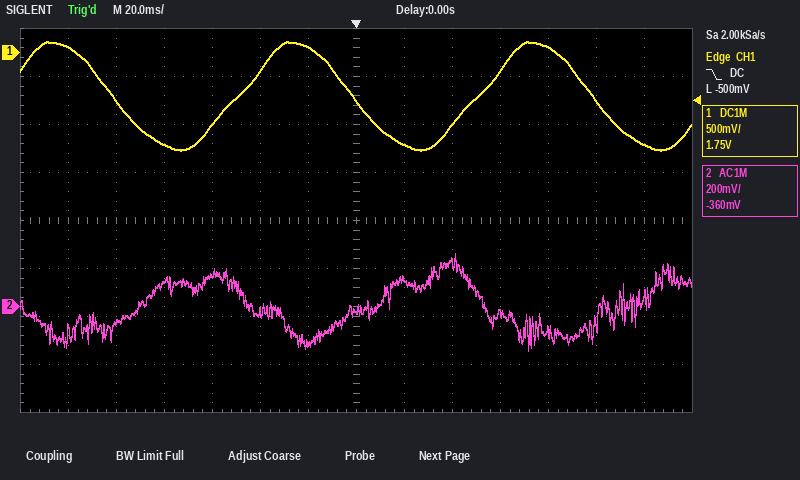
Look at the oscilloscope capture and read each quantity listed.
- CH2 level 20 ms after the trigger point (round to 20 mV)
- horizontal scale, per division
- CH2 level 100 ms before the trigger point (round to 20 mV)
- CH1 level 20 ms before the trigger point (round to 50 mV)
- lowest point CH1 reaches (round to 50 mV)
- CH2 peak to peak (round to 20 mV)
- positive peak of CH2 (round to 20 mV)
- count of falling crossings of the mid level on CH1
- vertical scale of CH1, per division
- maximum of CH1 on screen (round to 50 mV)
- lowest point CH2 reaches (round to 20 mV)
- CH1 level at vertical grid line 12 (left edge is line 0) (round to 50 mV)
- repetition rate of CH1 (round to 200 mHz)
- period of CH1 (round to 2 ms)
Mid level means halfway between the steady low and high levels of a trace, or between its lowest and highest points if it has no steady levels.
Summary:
120 mV
20 ms
-60 mV
50 mV
-1.00 V
400 mV
220 mV
3
500 mV
100 mV
-180 mV
-500 mV
10.0 Hz
100 ms
